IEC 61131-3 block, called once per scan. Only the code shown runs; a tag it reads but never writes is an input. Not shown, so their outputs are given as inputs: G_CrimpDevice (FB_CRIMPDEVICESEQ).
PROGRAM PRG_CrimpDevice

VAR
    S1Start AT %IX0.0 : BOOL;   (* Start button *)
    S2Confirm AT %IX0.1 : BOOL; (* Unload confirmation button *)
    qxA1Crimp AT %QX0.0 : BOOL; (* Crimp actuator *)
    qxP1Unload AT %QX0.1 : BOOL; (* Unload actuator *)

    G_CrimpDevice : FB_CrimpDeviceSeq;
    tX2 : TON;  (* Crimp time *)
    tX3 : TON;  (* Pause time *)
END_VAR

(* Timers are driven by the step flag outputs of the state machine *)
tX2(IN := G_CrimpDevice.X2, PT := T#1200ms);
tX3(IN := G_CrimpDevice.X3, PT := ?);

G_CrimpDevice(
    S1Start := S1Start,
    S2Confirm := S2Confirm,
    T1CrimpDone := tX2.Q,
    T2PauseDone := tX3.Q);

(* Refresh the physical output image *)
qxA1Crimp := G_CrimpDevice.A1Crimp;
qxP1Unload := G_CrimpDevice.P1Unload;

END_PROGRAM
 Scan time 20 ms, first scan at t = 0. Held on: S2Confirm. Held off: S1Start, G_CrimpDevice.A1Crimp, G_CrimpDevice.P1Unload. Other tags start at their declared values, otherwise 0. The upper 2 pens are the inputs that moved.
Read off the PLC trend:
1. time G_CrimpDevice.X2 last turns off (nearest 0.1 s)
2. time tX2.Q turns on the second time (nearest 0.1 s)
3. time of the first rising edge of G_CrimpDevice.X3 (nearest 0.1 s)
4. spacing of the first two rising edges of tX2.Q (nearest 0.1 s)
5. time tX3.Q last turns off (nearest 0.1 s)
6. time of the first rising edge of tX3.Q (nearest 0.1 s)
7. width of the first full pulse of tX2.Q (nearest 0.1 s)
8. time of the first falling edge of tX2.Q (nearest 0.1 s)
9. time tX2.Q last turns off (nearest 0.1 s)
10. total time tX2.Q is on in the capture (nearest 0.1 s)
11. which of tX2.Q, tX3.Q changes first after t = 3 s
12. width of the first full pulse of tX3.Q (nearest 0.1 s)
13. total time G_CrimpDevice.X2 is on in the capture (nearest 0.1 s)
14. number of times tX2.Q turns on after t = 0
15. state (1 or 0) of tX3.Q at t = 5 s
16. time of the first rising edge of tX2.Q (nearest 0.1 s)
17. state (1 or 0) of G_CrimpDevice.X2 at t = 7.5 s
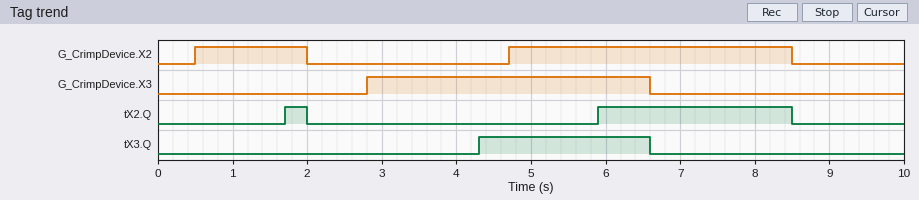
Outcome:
8.5 s
5.9 s
2.8 s
4.2 s
6.6 s
4.3 s
0.3 s
2.0 s
8.5 s
2.9 s
tX3.Q
2.3 s
5.3 s
2
1
1.7 s
1
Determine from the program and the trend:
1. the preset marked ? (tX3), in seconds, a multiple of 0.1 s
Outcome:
1.5 s
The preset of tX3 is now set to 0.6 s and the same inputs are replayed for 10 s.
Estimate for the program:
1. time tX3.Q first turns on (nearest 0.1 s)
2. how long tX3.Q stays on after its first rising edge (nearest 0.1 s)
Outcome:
3.4 s
3.2 s
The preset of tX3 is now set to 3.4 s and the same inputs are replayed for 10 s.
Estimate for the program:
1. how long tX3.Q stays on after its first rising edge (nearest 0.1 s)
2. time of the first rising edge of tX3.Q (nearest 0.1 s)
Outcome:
0.4 s
6.2 s
